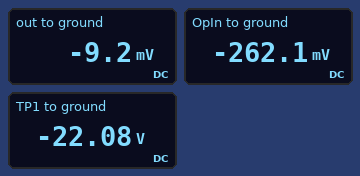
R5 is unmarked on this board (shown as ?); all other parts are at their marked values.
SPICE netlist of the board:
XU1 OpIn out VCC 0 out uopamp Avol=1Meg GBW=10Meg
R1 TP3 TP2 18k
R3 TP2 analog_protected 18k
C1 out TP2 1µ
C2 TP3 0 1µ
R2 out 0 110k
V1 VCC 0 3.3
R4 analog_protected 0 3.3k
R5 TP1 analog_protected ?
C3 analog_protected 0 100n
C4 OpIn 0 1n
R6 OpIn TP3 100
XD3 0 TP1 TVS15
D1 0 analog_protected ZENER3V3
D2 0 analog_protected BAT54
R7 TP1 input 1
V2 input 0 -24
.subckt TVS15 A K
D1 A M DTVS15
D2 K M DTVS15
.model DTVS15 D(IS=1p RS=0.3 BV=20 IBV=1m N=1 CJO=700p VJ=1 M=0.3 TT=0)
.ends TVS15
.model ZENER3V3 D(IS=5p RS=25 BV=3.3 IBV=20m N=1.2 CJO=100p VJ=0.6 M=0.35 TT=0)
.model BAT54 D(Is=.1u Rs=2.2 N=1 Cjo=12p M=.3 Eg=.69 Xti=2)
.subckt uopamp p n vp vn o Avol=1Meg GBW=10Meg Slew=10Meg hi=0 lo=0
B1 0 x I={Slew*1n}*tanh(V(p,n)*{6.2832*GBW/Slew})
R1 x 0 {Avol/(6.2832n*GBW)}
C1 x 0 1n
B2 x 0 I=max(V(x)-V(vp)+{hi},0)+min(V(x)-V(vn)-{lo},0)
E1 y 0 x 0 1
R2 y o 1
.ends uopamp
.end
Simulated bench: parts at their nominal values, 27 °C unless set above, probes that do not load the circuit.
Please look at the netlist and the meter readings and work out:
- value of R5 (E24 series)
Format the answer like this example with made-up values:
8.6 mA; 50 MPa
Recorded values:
10 kΩ
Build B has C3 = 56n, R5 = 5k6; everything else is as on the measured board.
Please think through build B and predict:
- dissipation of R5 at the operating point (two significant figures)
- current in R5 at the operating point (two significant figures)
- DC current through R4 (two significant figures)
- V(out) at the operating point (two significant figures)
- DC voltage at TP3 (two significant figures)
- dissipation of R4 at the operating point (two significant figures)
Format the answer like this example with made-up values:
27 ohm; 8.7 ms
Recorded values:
85 mW; 3.9 mA; 85 µA; -9.4 mV; -280 mV; 24 µW
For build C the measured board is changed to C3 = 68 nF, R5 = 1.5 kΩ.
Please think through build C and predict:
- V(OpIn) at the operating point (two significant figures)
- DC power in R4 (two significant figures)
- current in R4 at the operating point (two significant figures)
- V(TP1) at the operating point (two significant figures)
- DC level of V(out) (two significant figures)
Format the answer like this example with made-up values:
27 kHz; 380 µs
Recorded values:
-340 mV; 35 µW; 100 µA; -22 V; -9.7 mV
